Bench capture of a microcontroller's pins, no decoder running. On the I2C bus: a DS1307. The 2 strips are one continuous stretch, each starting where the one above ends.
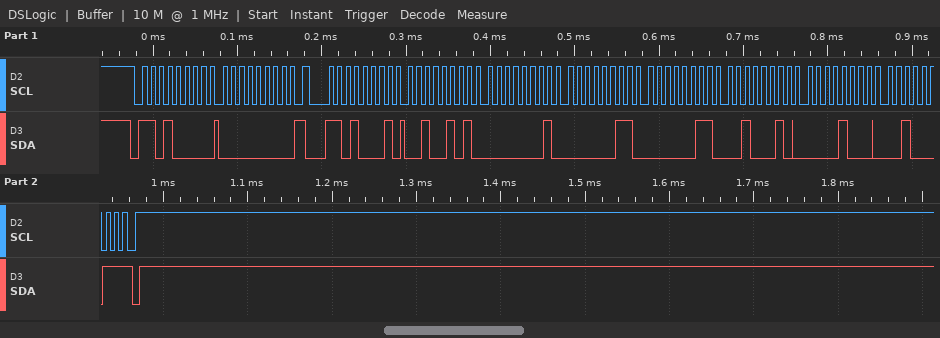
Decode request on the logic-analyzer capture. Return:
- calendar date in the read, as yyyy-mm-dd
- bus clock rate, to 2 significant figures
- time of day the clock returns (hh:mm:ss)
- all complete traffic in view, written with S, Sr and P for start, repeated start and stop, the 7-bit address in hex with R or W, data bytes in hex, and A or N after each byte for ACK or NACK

2023-08-22
100 kHz
03:01:25
S 68W A 00 A Sr 68R A 25 A 01 A 03 A 03 A 22 A 08 A 23 N P
